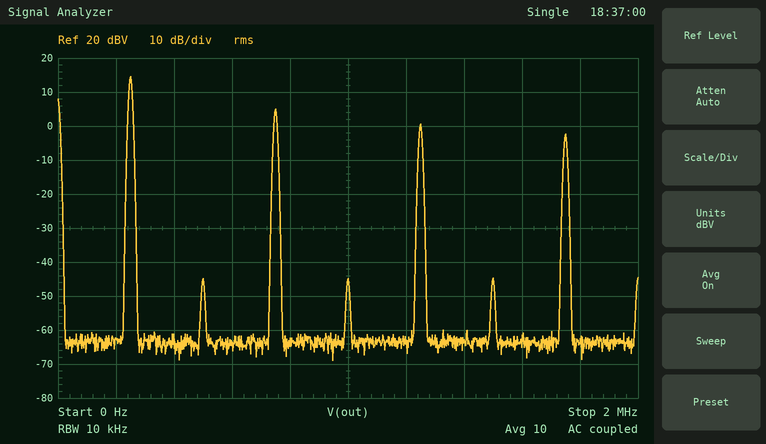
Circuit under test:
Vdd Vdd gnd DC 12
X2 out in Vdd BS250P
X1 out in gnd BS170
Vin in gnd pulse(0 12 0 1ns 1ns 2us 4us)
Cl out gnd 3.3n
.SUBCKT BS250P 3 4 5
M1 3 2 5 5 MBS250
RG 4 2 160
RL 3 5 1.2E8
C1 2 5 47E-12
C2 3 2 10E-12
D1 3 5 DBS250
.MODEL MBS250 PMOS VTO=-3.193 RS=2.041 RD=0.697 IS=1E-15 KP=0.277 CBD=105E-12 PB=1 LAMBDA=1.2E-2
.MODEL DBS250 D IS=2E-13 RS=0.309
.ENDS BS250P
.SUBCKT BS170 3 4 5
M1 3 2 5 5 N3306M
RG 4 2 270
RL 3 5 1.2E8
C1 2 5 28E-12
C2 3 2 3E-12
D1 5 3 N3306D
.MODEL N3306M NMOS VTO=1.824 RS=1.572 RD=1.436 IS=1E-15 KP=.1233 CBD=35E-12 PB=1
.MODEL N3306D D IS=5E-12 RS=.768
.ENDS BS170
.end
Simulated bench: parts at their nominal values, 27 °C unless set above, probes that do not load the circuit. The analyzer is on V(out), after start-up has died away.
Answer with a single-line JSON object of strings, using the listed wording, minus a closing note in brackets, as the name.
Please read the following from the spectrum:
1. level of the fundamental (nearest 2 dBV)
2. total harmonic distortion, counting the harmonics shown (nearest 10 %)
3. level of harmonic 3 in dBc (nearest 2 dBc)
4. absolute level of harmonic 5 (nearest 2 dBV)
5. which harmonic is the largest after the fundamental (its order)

{"level of the fundamental": "14 dBV", "total harmonic distortion, counting the harmonics shown": "40 %", "level of harmonic 3 in dBc": "-10 dBc", "absolute level of harmonic 5": "0 dBV", "which harmonic is the largest after the fundamental": "3"}
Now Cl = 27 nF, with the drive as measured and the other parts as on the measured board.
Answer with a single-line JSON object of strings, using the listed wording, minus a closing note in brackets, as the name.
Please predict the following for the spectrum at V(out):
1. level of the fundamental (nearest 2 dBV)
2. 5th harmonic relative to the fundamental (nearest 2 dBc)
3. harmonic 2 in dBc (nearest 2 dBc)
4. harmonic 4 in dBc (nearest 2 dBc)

{"level of the fundamental": "14 dBV", "5th harmonic relative to the fundamental": "-16 dBc", "harmonic 2 in dBc": "-42 dBc", "harmonic 4 in dBc": "-44 dBc"}
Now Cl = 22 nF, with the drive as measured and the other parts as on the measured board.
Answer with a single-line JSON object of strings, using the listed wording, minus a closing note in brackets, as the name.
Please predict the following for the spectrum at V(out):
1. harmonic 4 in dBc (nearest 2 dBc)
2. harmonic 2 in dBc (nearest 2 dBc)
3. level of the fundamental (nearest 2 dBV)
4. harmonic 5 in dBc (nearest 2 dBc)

{"harmonic 4 in dBc": "-46 dBc", "harmonic 2 in dBc": "-44 dBc", "level of the fundamental": "14 dBV", "harmonic 5 in dBc": "-16 dBc"}
